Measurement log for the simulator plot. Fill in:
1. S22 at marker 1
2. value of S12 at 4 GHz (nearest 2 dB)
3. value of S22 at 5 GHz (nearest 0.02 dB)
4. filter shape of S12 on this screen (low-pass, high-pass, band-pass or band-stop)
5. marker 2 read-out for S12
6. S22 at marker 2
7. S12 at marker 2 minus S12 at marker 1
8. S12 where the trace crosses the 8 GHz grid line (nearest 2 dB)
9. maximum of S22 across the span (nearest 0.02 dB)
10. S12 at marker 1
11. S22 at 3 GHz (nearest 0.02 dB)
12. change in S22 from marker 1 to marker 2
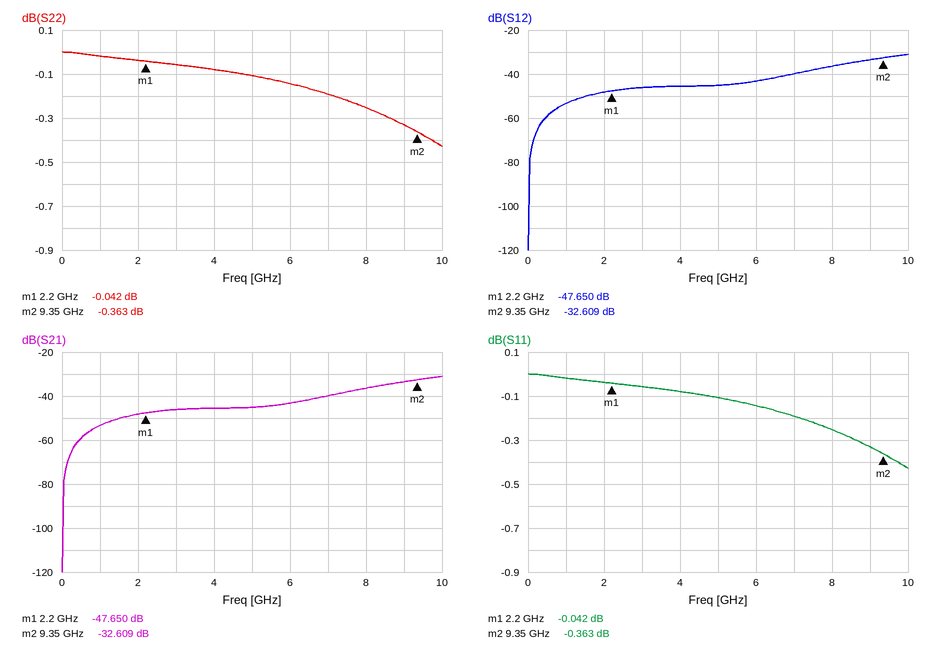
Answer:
-0.042 dB
-46 dB
-0.10 dB
high-pass
-32.609 dB
-0.363 dB
15.041 dB
-36 dB
0.00 dB
-47.650 dB
-0.06 dB
-0.321 dB
